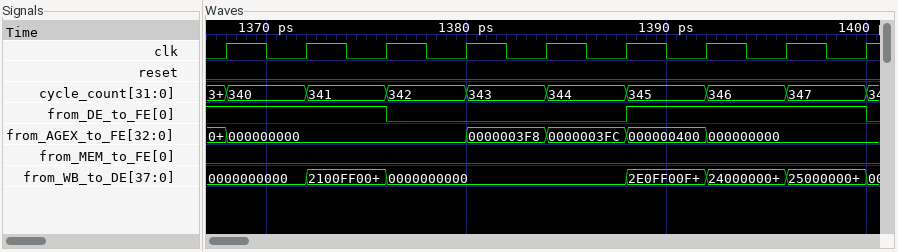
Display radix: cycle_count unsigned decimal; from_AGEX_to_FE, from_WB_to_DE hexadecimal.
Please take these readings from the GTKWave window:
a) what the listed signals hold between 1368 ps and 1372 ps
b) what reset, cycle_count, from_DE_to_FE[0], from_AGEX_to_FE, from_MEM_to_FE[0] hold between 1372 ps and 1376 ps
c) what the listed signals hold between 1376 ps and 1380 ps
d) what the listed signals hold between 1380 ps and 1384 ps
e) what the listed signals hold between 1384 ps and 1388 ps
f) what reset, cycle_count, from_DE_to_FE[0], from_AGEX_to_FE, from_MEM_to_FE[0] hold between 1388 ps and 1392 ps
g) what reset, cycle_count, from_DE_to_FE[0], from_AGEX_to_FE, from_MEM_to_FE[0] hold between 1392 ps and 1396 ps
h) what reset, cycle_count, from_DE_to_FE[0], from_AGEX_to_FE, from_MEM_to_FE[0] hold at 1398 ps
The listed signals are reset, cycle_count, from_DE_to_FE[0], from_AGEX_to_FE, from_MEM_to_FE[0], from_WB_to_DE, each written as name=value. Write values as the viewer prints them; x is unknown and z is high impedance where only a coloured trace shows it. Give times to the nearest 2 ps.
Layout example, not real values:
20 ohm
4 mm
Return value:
reset=0, cycle_count=340, from_DE_to_FE[0]=1, from_AGEX_to_FE=000000000, from_MEM_to_FE[0]=0, from_WB_to_DE=0000000000
reset=0, cycle_count=341, from_DE_to_FE[0]=1, from_AGEX_to_FE=000000000, from_MEM_to_FE[0]=0
reset=0, cycle_count=342, from_DE_to_FE[0]=0, from_AGEX_to_FE=000000000, from_MEM_to_FE[0]=0, from_WB_to_DE=0000000000
reset=0, cycle_count=343, from_DE_to_FE[0]=0, from_AGEX_to_FE=0000003F8, from_MEM_to_FE[0]=0, from_WB_to_DE=0000000000
reset=0, cycle_count=344, from_DE_to_FE[0]=0, from_AGEX_to_FE=0000003FC, from_MEM_to_FE[0]=0, from_WB_to_DE=0000000000
reset=0, cycle_count=345, from_DE_to_FE[0]=1, from_AGEX_to_FE=000000400, from_MEM_to_FE[0]=0
reset=0, cycle_count=346, from_DE_to_FE[0]=1, from_AGEX_to_FE=000000000, from_MEM_to_FE[0]=0
reset=0, cycle_count=347, from_DE_to_FE[0]=1, from_AGEX_to_FE=000000000, from_MEM_to_FE[0]=0
